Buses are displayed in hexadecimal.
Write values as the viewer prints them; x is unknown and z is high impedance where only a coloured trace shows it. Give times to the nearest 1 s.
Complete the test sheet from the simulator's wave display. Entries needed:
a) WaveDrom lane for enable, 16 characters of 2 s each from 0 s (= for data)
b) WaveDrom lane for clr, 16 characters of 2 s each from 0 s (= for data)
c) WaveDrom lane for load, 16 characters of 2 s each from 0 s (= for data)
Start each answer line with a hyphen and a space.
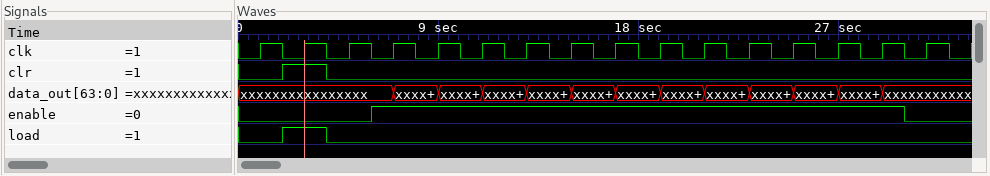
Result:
- {name: 'enable', wave: '0..1...........0'}
- {name: 'clr', wave: '010.............'}
- {name: 'load', wave: '010.............'}
